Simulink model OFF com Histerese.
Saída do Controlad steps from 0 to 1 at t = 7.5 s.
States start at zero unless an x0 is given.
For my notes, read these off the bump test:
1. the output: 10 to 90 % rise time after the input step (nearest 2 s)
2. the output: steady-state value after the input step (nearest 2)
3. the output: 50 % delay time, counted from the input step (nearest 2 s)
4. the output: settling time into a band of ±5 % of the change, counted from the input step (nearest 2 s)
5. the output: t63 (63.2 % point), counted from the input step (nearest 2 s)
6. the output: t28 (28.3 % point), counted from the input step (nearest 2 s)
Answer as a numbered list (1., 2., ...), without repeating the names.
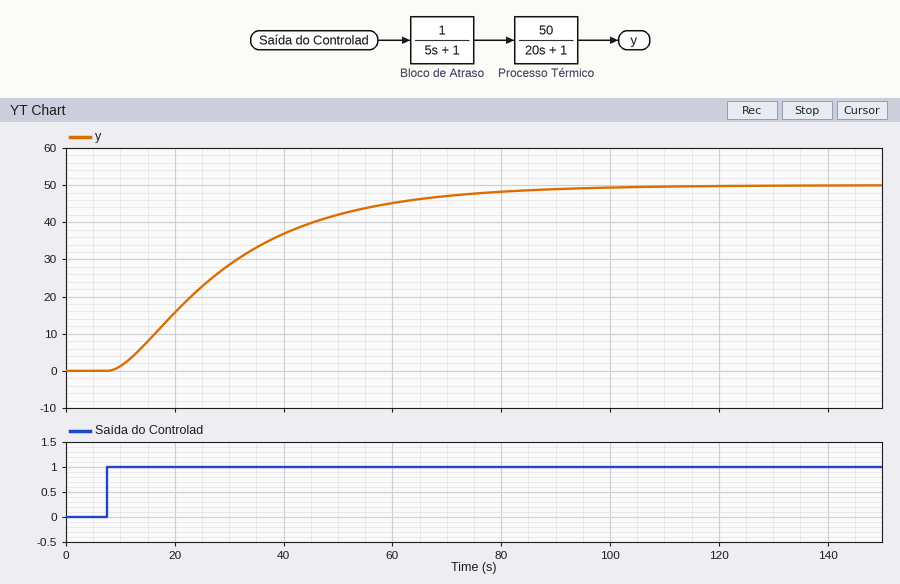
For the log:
1. 46 s
2. 50
3. 20 s
4. 66 s
5. 26 s
6. 12 s
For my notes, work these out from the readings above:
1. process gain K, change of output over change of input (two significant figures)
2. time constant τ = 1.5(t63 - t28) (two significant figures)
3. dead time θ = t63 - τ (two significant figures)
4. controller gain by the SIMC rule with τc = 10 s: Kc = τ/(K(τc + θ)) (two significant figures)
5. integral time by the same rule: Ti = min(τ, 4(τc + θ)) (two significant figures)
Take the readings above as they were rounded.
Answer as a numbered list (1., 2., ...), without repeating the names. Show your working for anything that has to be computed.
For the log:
1. (50 - 0) / 1 = 50
2. 1.5 × (26 - 12) = 21 s
3. 26 - 21 = 5.0 s
4. 21 / (50 × (10 + 5)) = 0.028
5. min(21, 4 × (10 + 5)) = 21 s
